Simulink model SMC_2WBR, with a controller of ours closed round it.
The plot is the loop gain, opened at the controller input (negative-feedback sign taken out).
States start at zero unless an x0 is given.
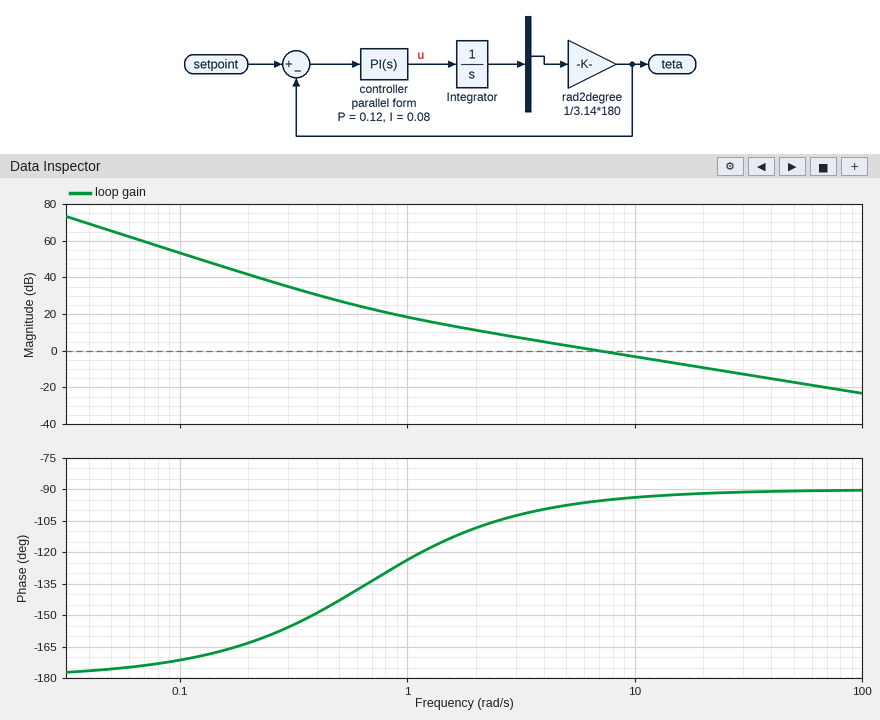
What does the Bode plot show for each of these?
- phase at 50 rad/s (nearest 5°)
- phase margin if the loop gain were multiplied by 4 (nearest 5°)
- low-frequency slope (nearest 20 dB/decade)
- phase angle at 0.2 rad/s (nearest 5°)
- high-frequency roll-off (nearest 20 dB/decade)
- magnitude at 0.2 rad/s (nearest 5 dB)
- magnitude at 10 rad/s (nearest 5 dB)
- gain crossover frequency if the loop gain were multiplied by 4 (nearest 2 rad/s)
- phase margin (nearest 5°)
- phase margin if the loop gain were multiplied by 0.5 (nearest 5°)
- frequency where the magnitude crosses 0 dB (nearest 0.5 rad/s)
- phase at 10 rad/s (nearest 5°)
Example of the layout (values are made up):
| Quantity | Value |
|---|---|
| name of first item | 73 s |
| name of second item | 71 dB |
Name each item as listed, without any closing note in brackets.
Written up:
| Quantity | Value |
|---|---|
| phase at 50 rad/s | -90° |
| phase margin if the loop gain were multiplied by 4 | 90° |
| low-frequency slope | -40 dB/decade |
| phase angle at 0.2 rad/s | -165° |
| high-frequency roll-off | -20 dB/decade |
| magnitude at 0.2 rad/s | 40 dB |
| magnitude at 10 rad/s | -5 dB |
| gain crossover frequency if the loop gain were multiplied by 4 | 28 rad/s |
| phase margin | 85° |
| phase margin if the loop gain were multiplied by 0.5 | 80° |
| frequency where the magnitude crosses 0 dB | 7.0 rad/s |
| phase at 10 rad/s | -95° |
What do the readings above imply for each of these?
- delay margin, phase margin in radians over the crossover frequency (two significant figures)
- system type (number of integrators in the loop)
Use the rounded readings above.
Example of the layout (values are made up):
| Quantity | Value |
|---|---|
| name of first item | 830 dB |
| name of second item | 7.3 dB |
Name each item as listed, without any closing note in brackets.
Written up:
| Quantity | Value |
|---|---|
| delay margin, phase margin in radians over the crossover frequency | 0.21 s |
| system type | 2 |
